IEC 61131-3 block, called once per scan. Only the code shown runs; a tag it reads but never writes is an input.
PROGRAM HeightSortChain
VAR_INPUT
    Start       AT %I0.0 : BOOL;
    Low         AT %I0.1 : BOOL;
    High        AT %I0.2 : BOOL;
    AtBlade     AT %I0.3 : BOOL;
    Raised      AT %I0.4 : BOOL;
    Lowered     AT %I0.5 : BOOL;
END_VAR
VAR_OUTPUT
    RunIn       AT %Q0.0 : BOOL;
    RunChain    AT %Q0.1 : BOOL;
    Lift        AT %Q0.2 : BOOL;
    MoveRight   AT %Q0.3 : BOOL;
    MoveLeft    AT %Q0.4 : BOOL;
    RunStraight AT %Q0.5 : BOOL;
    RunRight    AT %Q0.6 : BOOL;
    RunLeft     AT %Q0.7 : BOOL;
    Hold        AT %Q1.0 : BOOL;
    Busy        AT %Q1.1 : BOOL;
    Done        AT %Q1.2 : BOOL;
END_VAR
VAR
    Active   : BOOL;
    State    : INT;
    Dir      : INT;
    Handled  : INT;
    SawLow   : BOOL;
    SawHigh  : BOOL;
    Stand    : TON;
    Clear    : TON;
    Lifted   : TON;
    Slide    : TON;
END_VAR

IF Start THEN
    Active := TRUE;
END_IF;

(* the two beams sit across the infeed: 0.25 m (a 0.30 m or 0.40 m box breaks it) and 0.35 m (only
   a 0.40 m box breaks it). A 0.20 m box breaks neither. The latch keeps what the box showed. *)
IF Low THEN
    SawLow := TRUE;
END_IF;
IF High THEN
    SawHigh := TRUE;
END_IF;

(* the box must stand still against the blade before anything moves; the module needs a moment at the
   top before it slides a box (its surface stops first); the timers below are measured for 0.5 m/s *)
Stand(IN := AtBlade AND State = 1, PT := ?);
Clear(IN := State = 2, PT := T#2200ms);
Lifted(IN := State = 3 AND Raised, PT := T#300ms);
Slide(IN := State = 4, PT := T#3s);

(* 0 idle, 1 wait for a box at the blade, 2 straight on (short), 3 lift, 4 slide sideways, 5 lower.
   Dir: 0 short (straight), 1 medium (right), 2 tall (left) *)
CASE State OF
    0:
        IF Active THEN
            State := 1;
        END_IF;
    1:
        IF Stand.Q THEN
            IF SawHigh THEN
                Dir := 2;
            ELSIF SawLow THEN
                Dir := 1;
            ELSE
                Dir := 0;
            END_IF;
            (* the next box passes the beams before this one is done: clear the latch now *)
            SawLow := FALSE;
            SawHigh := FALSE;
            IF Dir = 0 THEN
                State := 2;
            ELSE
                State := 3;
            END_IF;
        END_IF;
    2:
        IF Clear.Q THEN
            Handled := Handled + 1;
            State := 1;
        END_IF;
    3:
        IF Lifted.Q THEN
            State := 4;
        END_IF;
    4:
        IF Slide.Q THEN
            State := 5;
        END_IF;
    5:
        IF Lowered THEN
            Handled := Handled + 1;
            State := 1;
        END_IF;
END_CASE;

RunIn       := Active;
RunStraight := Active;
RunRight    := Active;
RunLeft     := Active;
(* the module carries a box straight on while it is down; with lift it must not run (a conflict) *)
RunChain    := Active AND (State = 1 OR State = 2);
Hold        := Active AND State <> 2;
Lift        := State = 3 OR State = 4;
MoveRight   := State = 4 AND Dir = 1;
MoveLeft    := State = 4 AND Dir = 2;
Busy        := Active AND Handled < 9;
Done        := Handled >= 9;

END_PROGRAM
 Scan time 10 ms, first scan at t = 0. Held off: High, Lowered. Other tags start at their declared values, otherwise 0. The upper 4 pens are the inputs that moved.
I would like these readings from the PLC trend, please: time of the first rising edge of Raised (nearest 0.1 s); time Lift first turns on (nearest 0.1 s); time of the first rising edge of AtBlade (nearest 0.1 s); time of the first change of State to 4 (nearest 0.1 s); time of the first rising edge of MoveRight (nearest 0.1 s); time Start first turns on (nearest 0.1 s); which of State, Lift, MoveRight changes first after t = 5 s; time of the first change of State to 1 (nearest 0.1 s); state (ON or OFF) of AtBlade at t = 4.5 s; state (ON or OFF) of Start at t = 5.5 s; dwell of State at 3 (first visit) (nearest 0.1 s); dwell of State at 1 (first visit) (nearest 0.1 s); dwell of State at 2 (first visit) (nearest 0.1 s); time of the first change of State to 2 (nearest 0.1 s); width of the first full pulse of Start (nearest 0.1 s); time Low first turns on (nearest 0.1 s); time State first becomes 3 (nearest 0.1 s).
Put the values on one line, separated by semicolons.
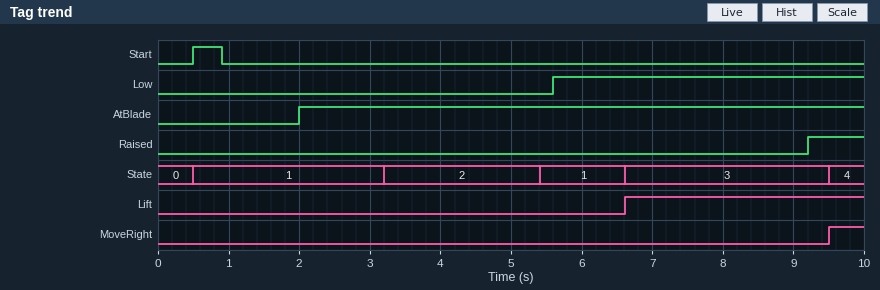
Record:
9.2 s; 6.6 s; 2.0 s; 9.5 s; 9.5 s; 0.5 s; State; 0.5 s; ON; OFF; 2.9 s; 2.7 s; 2.2 s; 3.2 s; 0.4 s; 5.6 s; 6.6 s
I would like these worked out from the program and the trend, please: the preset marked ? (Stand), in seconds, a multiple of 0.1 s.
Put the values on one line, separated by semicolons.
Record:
1.2 s
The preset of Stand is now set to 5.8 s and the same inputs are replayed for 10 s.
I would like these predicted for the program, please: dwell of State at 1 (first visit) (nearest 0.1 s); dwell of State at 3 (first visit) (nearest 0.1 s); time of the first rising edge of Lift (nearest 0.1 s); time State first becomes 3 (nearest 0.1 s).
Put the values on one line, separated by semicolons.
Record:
7.3 s; 1.7 s; 7.8 s; 7.8 s
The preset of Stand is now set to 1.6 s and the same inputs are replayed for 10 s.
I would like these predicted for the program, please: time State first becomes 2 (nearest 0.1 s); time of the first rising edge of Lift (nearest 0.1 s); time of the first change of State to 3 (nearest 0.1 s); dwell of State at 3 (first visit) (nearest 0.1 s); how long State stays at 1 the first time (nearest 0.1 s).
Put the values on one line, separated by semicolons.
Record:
3.6 s; 7.4 s; 7.4 s; 2.1 s; 3.1 s
